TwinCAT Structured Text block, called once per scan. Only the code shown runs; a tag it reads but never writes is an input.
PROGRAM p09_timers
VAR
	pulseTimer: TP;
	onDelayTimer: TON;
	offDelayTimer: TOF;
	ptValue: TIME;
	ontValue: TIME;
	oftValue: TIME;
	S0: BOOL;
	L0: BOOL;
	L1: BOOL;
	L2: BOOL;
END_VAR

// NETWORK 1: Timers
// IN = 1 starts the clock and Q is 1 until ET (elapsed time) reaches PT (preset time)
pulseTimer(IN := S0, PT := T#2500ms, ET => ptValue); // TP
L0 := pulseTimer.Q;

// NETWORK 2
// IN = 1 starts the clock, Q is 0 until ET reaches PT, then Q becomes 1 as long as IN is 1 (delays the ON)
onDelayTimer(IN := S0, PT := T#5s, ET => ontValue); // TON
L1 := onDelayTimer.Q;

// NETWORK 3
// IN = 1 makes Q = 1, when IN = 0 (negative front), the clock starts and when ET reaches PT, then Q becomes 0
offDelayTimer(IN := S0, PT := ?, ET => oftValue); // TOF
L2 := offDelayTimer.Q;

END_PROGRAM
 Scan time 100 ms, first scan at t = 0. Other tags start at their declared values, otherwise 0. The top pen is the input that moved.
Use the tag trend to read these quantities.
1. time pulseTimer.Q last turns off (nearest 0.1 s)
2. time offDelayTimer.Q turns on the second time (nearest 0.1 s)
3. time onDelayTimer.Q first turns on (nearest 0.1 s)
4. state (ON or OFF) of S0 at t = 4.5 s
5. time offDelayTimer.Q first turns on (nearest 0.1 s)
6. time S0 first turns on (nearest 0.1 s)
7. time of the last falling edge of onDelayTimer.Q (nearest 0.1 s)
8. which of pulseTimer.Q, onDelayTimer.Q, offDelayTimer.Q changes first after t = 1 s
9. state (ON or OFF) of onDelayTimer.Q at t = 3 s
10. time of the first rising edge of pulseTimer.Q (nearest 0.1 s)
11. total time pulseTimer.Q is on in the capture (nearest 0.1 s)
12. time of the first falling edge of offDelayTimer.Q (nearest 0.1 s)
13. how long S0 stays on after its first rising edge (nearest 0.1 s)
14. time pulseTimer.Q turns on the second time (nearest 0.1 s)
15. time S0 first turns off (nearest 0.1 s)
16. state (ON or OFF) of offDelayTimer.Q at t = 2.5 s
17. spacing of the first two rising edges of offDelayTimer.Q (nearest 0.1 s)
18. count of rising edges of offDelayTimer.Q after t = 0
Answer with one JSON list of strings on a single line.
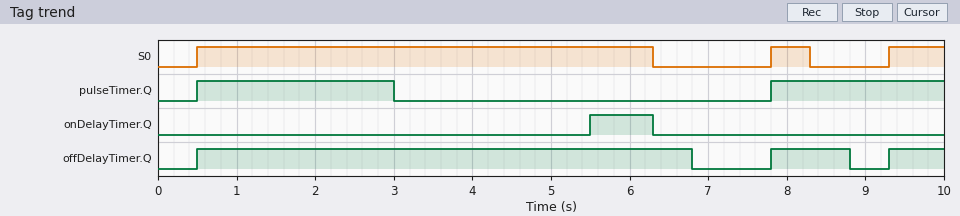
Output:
["3.0 s", "7.8 s", "5.5 s", "ON", "0.5 s", "0.5 s", "6.3 s", "pulseTimer.Q", "OFF", "0.5 s", "4.7 s", "6.8 s", "5.8 s", "7.8 s", "6.3 s", "ON", "7.3 s", "3"]
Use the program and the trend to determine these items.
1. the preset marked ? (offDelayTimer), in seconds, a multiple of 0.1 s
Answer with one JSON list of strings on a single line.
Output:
["0.5 s"]
